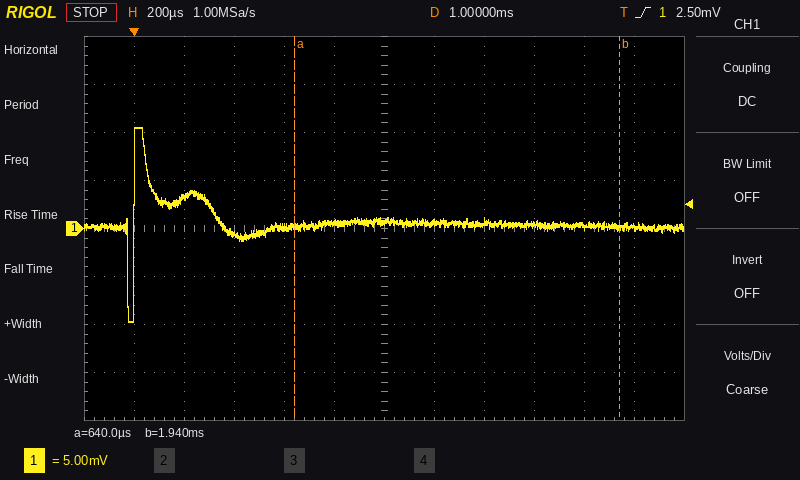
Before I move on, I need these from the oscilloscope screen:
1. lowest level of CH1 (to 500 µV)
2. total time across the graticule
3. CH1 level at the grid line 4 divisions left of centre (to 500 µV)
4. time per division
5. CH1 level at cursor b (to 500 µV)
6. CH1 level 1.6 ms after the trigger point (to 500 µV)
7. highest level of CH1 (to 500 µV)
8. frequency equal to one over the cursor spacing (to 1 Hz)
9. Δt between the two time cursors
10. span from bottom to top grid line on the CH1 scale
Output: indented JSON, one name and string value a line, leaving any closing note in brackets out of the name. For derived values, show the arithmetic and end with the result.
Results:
{
  "lowest level of CH1": "-9.5 mV",
  "total time across the graticule": "2.4 ms",
  "CH1 level at the grid line 4 divisions left of centre": "3.5 mV",
  "time per division": "200 µs",
  "CH1 level at cursor b": "0.0 mV",
  "CH1 level 1.6 ms after the trigger point": "500 µV",
  "highest level of CH1": "10.5 mV",
  "frequency equal to one over the cursor spacing": "1 / 1.30 ms ≈ 769 Hz",
  "Δt between the two time cursors": "1.94 ms − (640 µs) = 1.30 ms",
  "span from bottom to top grid line on the CH1 scale": "40 mV"
}
